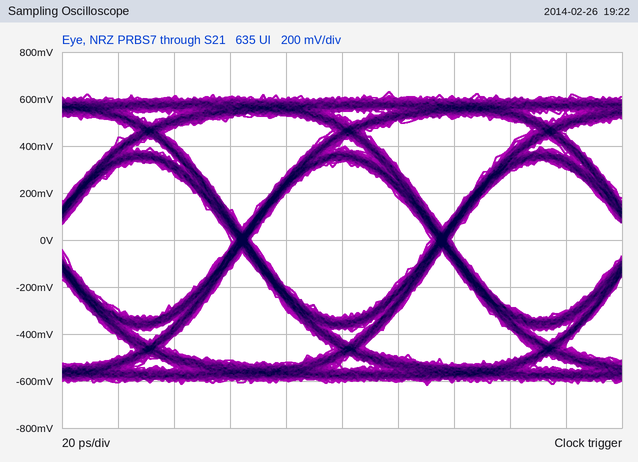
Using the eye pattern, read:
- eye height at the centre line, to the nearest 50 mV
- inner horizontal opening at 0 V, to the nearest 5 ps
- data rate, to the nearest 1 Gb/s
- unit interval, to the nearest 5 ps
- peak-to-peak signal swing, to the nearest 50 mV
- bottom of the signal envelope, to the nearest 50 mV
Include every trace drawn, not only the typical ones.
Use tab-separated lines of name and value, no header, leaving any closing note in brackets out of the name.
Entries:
eye height at the centre line, to the nearest 50 mV	650 mV
inner horizontal opening at 0 V, to the nearest 5 ps	65 ps
data rate, to the nearest 1 Gb/s	14 Gb/s
unit interval, to the nearest 5 ps	70 ps
peak-to-peak signal swing, to the nearest 50 mV	1.25 V
bottom of the signal envelope, to the nearest 50 mV	-600 mV
